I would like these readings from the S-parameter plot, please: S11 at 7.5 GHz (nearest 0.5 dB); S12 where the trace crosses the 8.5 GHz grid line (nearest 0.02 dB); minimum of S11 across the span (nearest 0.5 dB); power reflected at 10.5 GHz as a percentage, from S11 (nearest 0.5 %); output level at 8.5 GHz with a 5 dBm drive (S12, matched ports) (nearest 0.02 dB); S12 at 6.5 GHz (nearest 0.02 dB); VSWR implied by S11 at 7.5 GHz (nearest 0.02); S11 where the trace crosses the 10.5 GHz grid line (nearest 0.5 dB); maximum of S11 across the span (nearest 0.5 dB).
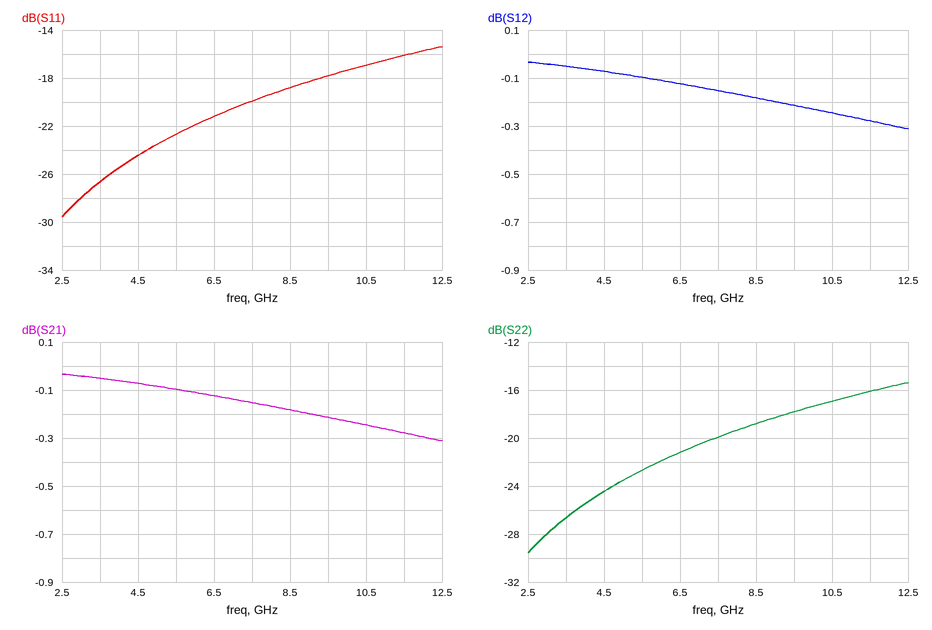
-20.0 dB
-0.18 dB
-29.5 dB
2.0 %
4.82 dBm
-0.12 dB
1.22
-17.0 dB
-15.5 dB
